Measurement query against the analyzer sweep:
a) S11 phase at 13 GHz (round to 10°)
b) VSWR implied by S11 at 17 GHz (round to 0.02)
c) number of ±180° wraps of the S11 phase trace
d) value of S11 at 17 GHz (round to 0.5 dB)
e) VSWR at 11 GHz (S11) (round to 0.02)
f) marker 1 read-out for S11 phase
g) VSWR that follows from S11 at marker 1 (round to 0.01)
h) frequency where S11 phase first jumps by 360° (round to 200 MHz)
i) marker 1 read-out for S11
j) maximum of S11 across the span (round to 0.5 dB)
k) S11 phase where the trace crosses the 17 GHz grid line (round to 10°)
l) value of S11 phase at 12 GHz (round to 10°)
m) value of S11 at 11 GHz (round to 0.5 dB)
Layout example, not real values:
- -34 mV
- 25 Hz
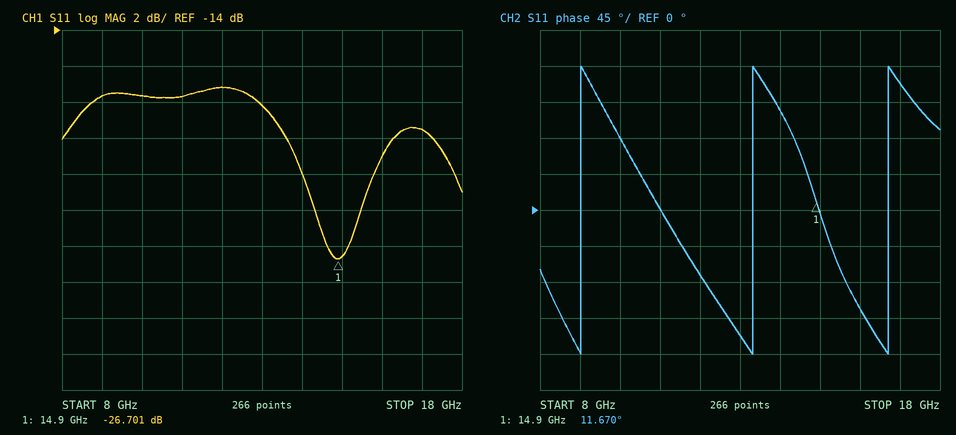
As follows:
- -160°
- 1.24
- 3
- -19.5 dB
- 1.30
- 11.670°
- 1.10
- 9.0 GHz
- -26.701 dB
- -17.0 dB
- 160°
- -80°
- -17.5 dB
